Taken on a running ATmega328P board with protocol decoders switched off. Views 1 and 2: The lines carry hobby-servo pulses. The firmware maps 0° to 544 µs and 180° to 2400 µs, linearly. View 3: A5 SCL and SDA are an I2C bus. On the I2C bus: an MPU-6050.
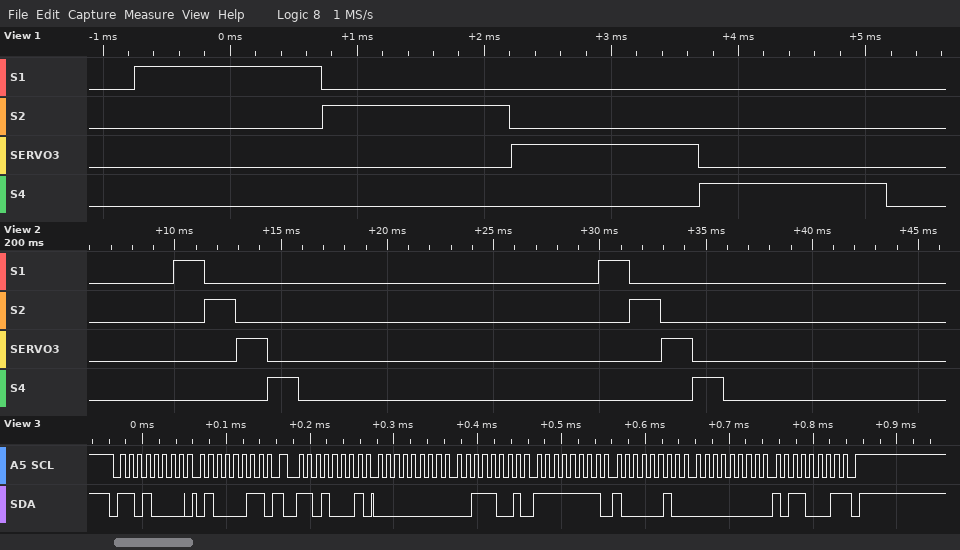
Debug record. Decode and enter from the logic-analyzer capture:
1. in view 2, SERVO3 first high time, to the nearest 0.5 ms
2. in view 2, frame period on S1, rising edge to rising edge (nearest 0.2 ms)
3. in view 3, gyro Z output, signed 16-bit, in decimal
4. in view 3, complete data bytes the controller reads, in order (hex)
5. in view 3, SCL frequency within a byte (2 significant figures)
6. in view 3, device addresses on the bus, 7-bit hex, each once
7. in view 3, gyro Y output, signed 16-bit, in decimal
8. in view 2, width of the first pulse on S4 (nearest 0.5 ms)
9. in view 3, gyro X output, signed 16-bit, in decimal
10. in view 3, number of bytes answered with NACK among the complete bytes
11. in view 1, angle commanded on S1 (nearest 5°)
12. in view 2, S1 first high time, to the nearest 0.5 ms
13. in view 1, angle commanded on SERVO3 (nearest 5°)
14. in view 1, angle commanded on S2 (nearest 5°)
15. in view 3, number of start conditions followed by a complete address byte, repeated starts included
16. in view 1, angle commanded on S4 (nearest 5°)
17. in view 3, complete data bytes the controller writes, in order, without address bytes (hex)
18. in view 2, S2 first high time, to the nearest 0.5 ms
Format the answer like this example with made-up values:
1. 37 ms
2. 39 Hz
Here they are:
1. 1.5 ms
2. 20.0 ms
3. 177
4. 00 39 FF 82 00 B1
5. 100 kHz
6. 0x68
7. -126
8. 1.5 ms
9. 57
10. 1
11. 90°
12. 1.5 ms
13. 90°
14. 90°
15. 2
16. 90°
17. 43
18. 1.5 ms
